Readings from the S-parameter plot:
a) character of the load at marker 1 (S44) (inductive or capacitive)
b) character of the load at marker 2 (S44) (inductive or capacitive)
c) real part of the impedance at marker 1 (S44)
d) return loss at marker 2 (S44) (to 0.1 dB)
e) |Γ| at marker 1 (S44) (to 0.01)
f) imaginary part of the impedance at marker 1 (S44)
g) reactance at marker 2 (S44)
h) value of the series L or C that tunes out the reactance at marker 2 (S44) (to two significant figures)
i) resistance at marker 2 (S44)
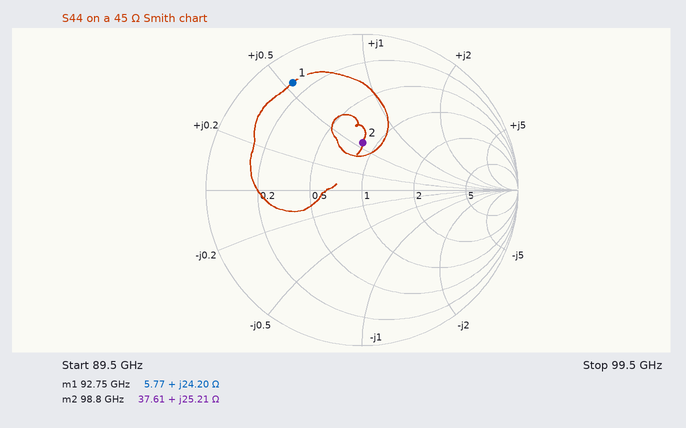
inductive
inductive
5.77 Ω
10.3 dB
0.82
+24.20 Ω
+25.21 Ω
64 fF
37.61 Ω
